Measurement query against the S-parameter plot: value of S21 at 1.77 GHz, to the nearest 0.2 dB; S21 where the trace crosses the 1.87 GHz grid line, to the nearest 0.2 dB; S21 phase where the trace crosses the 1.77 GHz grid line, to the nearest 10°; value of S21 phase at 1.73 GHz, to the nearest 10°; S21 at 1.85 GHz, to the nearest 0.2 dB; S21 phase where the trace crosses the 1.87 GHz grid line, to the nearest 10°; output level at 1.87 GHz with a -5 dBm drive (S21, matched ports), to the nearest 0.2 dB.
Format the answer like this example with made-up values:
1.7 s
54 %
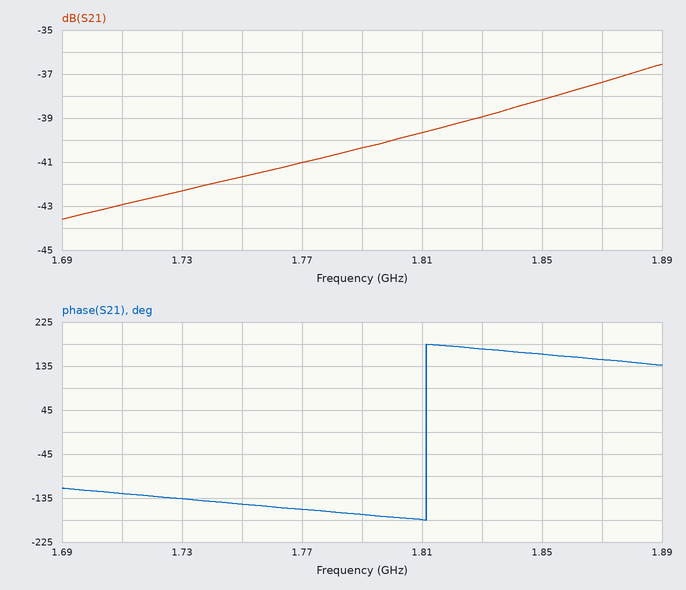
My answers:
-41.0 dB
-37.4 dB
-160°
-140°
-38.2 dB
150°
-42.4 dBm
